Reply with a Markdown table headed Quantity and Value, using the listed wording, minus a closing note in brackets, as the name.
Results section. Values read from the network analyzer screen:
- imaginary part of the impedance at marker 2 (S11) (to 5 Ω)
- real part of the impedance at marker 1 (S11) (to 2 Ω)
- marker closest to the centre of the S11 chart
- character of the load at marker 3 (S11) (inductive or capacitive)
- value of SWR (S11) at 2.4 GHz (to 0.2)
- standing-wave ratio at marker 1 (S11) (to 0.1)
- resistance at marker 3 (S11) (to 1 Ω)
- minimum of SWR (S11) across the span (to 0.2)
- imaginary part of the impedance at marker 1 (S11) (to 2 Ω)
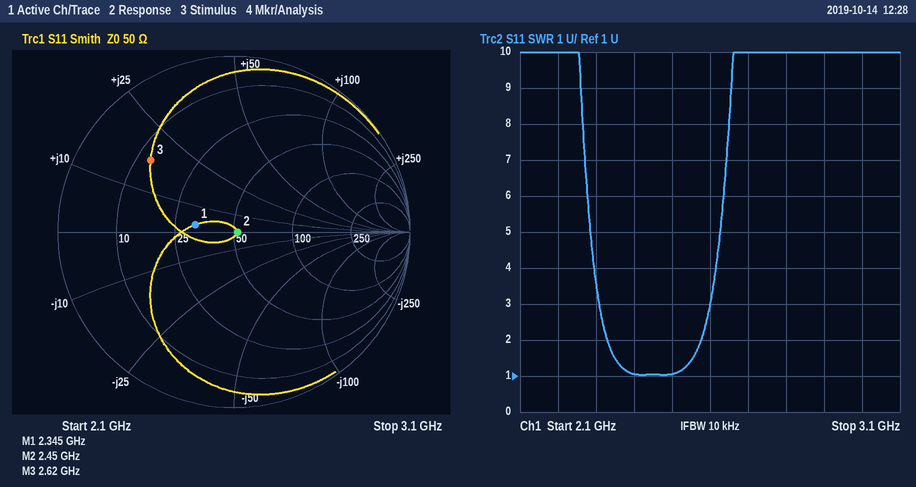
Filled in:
| Quantity | Value |
|---|---|
| imaginary part of the impedance at marker 2 (S11) | 0 Ω |
| real part of the impedance at marker 1 (S11) | 32 Ω |
| marker closest to the centre of the S11 chart | marker 2 |
| character of the load at marker 3 (S11) | inductive |
| value of SWR (S11) at 2.4 GHz | 1.0 |
| standing-wave ratio at marker 1 (S11) | 1.6 |
| resistance at marker 3 (S11) | 13 Ω |
| minimum of SWR (S11) across the span | 1.0 |
| imaginary part of the impedance at marker 1 (S11) | +2 Ω |
